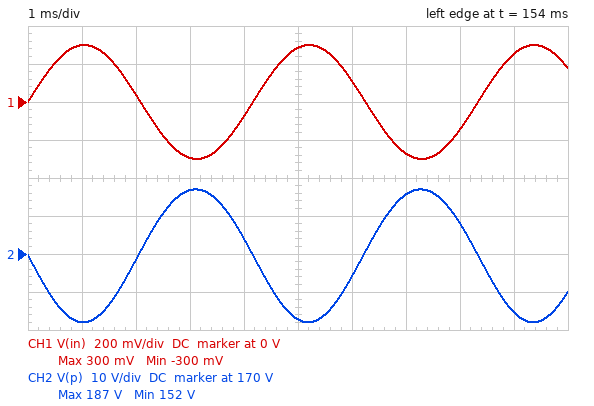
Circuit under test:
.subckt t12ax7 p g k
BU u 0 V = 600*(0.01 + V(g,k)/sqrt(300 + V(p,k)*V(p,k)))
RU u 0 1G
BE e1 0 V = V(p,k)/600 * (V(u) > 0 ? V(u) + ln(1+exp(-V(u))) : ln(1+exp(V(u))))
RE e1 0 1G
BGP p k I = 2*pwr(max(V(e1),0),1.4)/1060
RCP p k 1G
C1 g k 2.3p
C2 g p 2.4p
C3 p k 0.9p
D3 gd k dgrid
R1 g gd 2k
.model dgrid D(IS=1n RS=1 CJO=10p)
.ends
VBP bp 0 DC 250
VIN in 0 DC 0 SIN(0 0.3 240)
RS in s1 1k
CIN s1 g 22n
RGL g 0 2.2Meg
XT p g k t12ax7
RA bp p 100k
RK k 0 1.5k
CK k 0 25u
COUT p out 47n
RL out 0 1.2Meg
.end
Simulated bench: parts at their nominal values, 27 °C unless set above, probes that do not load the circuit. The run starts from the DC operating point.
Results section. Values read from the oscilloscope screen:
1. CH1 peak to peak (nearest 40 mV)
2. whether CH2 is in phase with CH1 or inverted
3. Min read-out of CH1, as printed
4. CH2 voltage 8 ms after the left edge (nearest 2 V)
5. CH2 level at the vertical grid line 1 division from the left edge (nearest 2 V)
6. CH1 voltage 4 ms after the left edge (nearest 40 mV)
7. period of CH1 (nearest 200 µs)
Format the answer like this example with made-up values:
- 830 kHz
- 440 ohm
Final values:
- 600 mV
- inverted
- -300 mV
- 178 V
- 152 V
- -80 mV
- 4.2 ms
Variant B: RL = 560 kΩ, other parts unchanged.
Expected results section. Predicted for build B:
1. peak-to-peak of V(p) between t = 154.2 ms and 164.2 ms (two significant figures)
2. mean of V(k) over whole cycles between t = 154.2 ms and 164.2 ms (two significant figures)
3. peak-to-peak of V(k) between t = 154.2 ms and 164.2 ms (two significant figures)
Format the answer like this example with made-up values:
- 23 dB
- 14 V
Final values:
- 34 V
- 1.2 V
- 11 mV
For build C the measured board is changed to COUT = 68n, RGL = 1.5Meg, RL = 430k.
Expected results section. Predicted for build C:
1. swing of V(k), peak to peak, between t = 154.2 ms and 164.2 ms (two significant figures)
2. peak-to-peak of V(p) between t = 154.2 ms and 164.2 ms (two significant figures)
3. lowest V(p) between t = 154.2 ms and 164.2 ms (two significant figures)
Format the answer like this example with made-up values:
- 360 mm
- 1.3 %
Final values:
- 11 mV
- 33 V
- 150 V
